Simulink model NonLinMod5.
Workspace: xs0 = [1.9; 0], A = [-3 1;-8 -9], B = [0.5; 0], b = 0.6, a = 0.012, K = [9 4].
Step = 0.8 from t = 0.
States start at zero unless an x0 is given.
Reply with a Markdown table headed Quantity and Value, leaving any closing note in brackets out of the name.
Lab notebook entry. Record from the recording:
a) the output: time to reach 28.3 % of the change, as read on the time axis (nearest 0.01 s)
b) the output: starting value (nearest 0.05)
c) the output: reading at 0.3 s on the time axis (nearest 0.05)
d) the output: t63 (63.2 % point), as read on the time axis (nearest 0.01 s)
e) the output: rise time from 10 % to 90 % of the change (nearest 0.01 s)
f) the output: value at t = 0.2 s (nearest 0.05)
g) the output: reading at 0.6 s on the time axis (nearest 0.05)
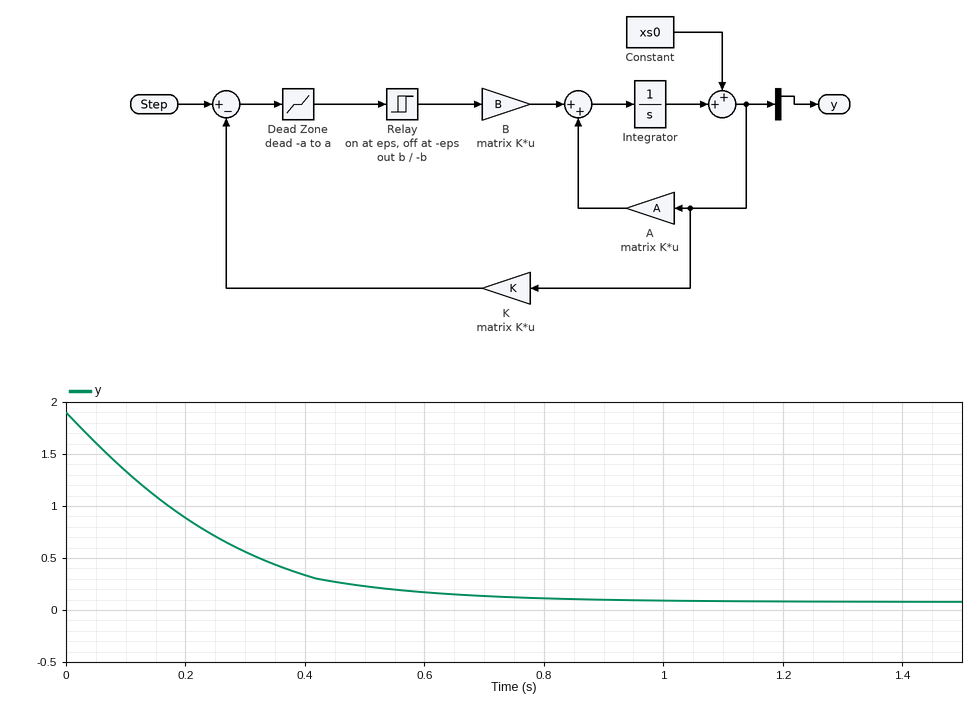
| Quantity | Value |
|---|---|
| the output: time to reach 28.3 % of the change, as read on the time axis | 0.09 s |
| the output: starting value | 1.90 |
| the output: reading at 0.3 s on the time axis | 0.55 |
| the output: t63 (63.2 % point), as read on the time axis | 0.24 s |
| the output: rise time from 10 % to 90 % of the change | 0.43 s |
| the output: value at t = 0.2 s | 0.90 |
| the output: reading at 0.6 s on the time axis | 0.15 |
